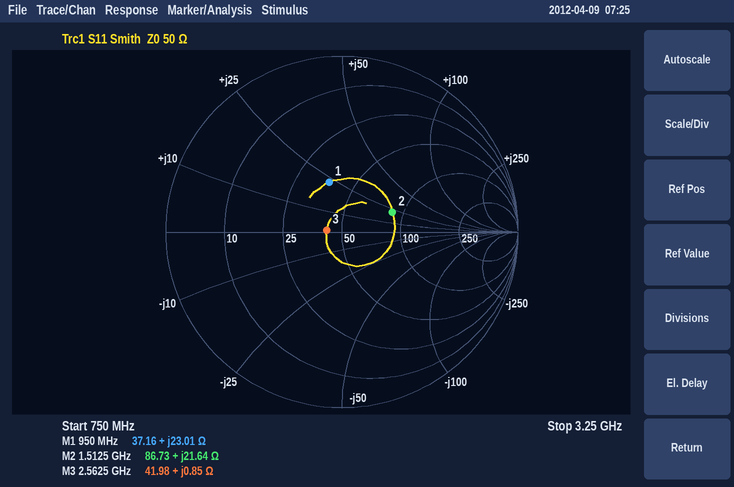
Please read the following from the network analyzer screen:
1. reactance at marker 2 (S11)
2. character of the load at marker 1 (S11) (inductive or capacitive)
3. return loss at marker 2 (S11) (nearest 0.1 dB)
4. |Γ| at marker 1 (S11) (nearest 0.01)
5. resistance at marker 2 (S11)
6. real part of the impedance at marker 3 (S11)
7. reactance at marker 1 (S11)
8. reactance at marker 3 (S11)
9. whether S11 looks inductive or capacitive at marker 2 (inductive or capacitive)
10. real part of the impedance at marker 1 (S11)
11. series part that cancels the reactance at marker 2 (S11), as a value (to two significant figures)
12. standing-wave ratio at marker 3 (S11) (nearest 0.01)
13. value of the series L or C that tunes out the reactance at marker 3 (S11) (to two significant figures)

+21.64 Ω
inductive
10.2 dB
0.29
86.73 Ω
41.98 Ω
+23.01 Ω
+0.85 Ω
inductive
37.16 Ω
4.9 pF
1.19
73 pF
